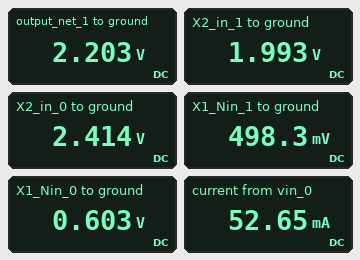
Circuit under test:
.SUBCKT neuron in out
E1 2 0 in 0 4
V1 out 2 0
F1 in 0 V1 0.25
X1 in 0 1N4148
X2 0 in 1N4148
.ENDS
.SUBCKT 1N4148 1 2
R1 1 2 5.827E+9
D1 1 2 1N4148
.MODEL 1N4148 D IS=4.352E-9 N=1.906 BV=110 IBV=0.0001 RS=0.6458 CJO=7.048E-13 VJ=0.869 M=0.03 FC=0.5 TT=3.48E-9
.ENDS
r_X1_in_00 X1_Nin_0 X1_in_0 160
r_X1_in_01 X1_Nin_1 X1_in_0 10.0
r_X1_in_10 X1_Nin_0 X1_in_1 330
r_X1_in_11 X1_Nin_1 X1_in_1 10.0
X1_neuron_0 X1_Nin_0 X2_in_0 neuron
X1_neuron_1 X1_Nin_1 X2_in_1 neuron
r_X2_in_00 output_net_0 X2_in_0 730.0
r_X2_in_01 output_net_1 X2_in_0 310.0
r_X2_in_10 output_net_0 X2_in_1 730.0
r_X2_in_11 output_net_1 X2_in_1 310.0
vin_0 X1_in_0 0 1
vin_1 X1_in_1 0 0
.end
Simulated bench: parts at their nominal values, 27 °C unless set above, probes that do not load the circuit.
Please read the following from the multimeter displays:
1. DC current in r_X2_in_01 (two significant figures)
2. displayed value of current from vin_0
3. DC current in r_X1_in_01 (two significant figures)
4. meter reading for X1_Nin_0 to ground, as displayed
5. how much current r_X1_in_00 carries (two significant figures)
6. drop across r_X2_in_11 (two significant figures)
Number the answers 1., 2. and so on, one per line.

1. 680 µA
2. 52.65 mA
3. 50 mA
4. 0.603 V
5. 2.5 mA
6. 210 mV
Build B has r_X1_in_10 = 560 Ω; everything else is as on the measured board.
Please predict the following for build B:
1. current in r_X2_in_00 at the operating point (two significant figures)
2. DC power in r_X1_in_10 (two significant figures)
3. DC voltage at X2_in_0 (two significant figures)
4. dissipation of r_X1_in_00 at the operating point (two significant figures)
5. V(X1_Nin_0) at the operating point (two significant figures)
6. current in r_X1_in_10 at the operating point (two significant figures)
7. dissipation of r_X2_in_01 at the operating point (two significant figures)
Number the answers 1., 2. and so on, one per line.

1. 360 µA
2. 710 µW
3. 2.5 V
4. 860 µW
5. 630 mV
6. 1.1 mA
7. 220 µW
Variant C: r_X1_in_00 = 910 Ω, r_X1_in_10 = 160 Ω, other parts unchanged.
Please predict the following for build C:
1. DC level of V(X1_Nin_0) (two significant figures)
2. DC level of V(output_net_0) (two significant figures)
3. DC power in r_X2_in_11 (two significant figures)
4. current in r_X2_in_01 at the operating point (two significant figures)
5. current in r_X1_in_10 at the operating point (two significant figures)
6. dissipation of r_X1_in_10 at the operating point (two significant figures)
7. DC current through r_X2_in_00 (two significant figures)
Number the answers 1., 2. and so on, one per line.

1. -12 mV
2. 990 mV
3. 3.5 mW
4. 3.3 mA
5. 77 µA
6. 950 nW
7. 1.4 mA
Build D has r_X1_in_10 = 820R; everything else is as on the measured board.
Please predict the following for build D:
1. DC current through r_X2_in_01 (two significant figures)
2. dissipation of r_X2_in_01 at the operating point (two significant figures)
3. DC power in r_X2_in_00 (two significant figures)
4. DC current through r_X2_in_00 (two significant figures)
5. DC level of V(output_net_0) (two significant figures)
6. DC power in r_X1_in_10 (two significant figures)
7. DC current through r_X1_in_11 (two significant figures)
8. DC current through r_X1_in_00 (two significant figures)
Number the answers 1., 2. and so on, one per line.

1. 910 µA
2. 260 µW
3. 110 µW
4. 390 µA
5. 2.3 V
6. 500 µW
7. 50 mA
8. 2.3 mA
